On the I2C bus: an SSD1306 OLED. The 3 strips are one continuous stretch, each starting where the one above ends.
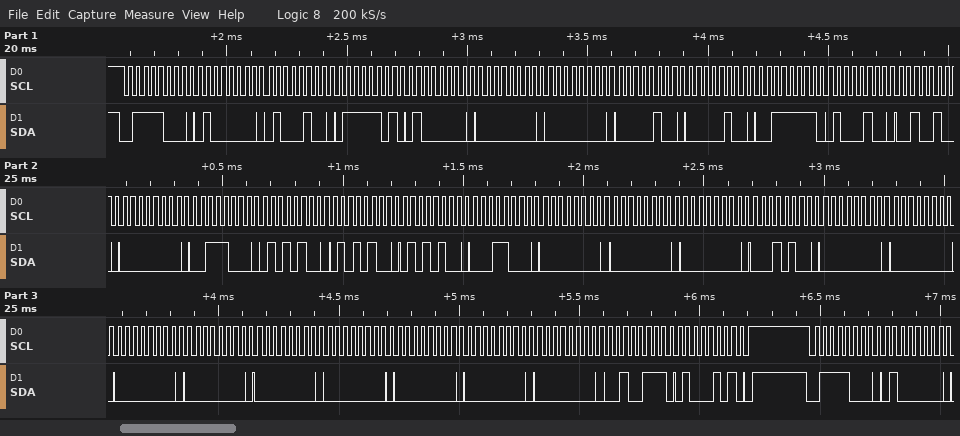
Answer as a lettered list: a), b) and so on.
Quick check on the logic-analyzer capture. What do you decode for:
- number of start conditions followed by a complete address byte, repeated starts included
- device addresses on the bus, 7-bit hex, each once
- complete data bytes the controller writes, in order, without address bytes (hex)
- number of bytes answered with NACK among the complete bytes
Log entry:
a) 2
b) 0x3C
c) 40 44 7D 40 00 00 04 04 3F 44 24 00 38 54 54 54 18 00 00 00 14 00 00 00 00 00 00 00 00 00 27 45 40
d) 0
